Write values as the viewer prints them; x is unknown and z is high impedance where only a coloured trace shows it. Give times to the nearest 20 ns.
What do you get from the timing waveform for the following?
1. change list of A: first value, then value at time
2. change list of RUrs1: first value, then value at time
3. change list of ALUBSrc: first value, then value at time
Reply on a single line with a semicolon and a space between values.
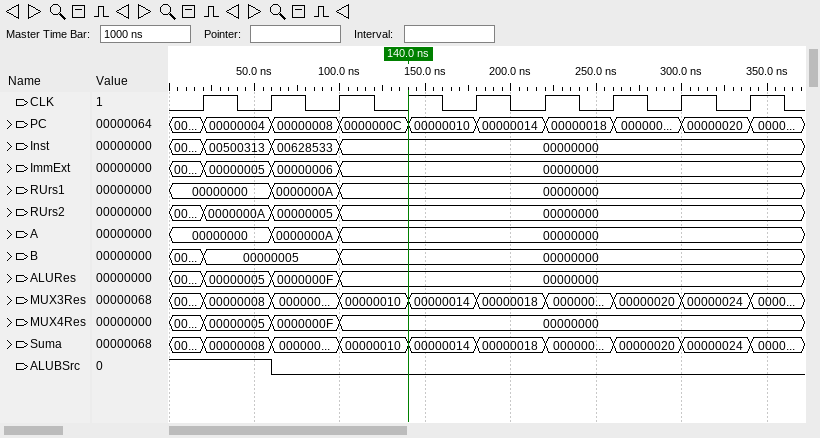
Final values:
00000000, 0000000A at 60 ns, 00000000 at 100 ns; 00000000, 0000000A at 60 ns, 00000000 at 100 ns; 1, 0 at 60 ns
